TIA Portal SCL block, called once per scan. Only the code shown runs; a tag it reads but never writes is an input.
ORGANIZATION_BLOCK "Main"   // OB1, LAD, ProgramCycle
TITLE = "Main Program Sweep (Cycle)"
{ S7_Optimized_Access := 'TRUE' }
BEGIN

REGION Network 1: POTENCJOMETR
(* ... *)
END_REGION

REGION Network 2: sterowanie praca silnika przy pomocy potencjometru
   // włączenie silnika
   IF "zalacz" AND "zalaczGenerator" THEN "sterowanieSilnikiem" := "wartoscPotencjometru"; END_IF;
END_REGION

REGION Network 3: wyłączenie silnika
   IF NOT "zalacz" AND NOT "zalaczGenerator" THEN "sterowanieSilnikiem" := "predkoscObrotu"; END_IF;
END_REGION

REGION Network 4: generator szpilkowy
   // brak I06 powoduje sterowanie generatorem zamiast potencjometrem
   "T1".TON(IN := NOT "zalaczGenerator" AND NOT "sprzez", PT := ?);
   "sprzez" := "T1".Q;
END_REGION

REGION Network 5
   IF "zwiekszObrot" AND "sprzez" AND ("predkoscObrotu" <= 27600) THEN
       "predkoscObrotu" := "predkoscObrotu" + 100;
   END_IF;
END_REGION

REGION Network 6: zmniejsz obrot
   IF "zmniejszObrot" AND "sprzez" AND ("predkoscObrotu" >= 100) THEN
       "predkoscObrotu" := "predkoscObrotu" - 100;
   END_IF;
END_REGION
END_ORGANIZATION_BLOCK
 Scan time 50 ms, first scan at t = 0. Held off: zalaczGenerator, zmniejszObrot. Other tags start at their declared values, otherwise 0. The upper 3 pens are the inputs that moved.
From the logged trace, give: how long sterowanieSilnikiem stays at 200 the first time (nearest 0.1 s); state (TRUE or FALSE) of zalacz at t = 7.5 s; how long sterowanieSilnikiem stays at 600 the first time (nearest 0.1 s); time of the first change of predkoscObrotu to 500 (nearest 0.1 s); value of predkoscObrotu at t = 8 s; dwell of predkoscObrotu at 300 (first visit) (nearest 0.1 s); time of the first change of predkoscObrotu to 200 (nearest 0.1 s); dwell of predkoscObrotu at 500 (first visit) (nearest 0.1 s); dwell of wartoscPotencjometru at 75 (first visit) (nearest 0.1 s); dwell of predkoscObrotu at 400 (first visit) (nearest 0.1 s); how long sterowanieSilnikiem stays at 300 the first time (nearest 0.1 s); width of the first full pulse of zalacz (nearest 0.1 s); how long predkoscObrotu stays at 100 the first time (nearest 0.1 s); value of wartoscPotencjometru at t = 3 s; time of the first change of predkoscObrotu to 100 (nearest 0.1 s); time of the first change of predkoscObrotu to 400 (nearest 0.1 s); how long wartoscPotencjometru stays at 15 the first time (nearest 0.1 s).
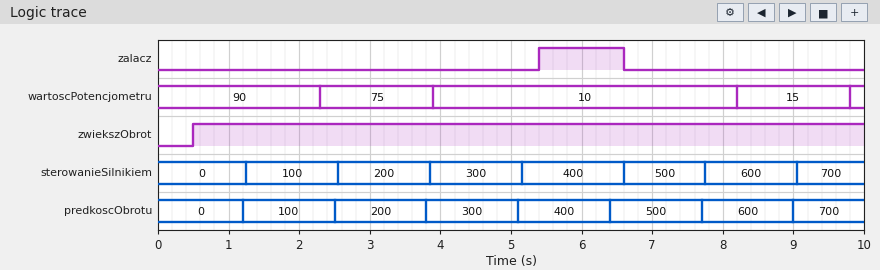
1.3 s
FALSE
1.3 s
6.4 s
600
1.3 s
2.5 s
1.3 s
1.6 s
1.3 s
1.3 s
1.2 s
1.3 s
75
1.2 s
5.1 s
1.6 s
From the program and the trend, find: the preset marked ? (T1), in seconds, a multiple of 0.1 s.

1.2 s
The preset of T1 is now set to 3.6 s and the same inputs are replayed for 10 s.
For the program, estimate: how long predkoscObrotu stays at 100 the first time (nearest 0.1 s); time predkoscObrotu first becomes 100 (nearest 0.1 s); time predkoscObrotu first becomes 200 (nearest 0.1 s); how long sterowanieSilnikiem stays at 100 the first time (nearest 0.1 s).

3.7 s
3.6 s
7.3 s
3.7 s
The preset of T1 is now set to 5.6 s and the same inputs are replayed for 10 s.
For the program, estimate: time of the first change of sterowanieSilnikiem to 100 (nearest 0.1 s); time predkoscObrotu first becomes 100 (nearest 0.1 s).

6.6 s
5.6 s
